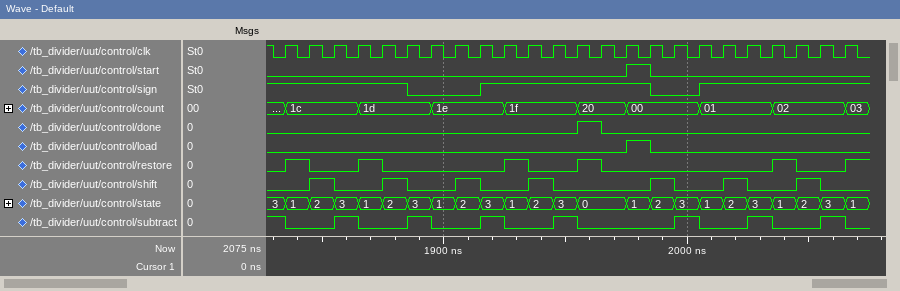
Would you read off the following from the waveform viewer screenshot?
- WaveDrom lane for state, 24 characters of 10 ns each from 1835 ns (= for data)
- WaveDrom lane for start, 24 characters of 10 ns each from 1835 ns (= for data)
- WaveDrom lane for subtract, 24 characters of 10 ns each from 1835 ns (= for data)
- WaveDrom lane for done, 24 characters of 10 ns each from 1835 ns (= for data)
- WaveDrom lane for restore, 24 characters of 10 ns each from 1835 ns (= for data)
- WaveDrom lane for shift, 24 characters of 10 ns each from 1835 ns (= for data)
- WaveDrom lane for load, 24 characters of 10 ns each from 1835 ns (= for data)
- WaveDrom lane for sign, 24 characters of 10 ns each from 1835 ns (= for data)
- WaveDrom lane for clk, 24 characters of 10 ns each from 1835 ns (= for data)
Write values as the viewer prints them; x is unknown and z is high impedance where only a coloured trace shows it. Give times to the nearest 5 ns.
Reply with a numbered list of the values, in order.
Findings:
1. {name: 'state', wave: '=============.==========', data: '1 2 3 1 2 3 1 2 3 1 2 3 0 1 2 3 1 2 3 1 2 3 1'}
2. {name: 'start', wave: '0.............10........'}
3. {name: 'subtract', wave: '0.10.10.10.10...10.10.10'}
4. {name: 'done', wave: '0...........10..........'}
5. {name: 'restore', wave: '10.10....10.10......10.1'}
6. {name: 'shift', wave: '010.10.10.10...10.10.10.'}
7. {name: 'load', wave: '0.............10........'}
8. {name: 'sign', wave: '1....0..1......0.1......'}
9. {name: 'clk', wave: 'p.......................'}
